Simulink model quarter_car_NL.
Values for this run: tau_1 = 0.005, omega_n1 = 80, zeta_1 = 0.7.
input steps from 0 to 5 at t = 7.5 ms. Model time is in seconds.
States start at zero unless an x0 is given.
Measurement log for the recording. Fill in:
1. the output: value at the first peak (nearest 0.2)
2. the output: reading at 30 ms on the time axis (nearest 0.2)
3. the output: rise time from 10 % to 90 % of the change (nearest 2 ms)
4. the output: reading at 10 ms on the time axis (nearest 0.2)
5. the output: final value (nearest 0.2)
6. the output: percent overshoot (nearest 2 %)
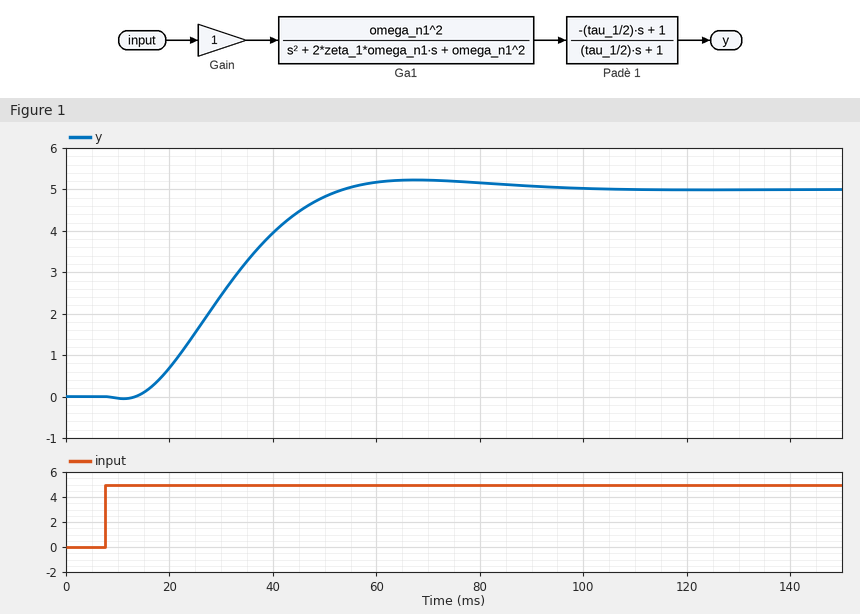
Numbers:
5.2
2.4
26 ms
0.0
5.0
4 %
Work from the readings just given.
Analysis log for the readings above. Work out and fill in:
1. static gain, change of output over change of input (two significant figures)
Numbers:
1.0
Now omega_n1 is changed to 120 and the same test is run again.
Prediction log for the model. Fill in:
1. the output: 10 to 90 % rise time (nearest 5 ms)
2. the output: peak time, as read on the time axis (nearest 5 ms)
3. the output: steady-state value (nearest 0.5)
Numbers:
20 ms
50 ms
5.0
